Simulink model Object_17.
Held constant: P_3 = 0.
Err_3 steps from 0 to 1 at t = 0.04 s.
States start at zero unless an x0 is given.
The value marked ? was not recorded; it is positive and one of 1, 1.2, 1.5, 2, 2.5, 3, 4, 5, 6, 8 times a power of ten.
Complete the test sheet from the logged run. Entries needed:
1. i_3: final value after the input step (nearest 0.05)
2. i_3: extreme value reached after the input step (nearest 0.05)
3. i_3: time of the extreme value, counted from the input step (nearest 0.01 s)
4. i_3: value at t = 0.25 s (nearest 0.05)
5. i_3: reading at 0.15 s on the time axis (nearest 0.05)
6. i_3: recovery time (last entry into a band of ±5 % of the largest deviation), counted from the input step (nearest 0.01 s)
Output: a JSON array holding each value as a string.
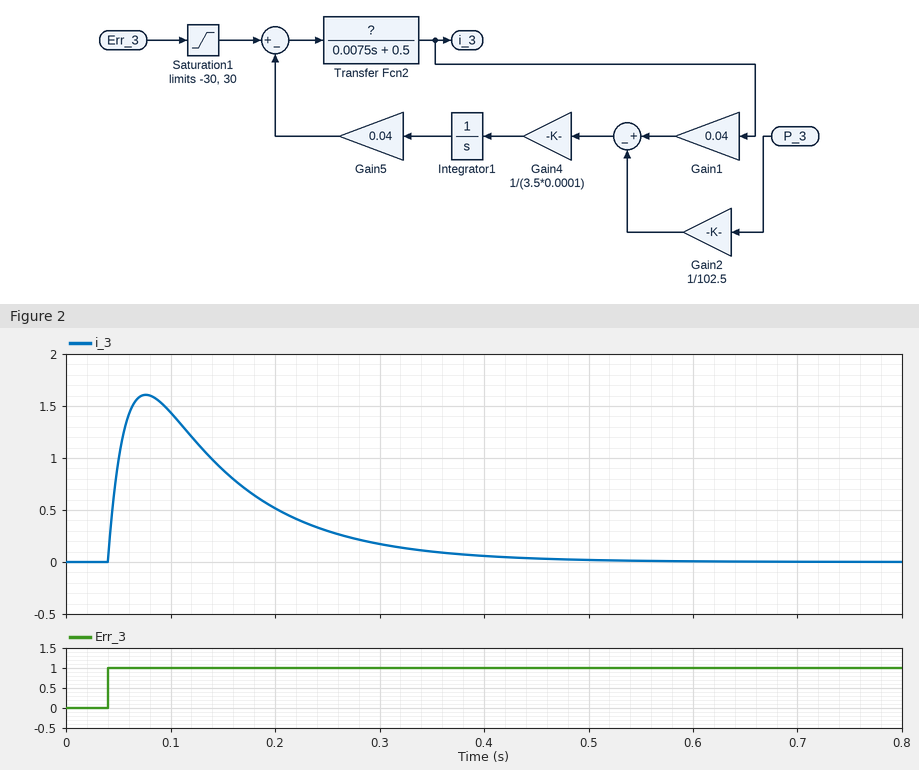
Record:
["0.00", "1.60", "0.04 s", "0.30", "0.90", "0.33 s"]
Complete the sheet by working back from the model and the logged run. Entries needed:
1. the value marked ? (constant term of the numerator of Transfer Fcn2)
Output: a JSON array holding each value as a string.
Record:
["1"]
